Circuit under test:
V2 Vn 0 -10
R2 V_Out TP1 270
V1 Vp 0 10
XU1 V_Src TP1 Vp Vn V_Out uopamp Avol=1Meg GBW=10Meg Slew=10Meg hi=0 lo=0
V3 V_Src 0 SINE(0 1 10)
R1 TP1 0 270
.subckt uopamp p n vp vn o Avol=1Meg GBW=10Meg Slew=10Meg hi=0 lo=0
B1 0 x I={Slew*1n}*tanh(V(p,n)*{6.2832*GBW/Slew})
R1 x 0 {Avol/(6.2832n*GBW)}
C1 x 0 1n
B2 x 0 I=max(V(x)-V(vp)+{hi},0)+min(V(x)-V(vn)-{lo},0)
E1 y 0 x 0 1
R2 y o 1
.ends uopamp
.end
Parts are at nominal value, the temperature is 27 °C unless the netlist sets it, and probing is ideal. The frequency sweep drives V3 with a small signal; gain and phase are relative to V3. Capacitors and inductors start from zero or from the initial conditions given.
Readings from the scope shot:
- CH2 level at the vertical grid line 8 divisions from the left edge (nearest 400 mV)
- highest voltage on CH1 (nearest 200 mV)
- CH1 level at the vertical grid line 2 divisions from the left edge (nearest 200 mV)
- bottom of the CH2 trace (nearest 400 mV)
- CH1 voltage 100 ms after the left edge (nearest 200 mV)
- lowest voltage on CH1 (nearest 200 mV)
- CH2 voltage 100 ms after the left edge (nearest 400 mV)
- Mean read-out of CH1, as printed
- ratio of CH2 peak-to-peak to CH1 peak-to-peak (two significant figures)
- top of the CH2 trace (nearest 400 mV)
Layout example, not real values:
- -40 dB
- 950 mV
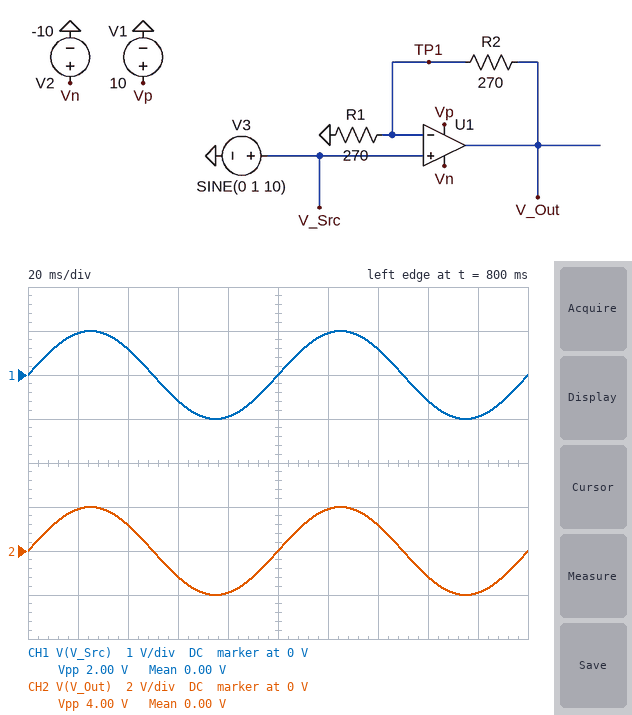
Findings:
- -1.2 V
- 1.0 V
- 600 mV
- -2.0 V
- 0 V
- -1.0 V
- 0 V
- 0.00 V
- 2.0
- 2.0 V
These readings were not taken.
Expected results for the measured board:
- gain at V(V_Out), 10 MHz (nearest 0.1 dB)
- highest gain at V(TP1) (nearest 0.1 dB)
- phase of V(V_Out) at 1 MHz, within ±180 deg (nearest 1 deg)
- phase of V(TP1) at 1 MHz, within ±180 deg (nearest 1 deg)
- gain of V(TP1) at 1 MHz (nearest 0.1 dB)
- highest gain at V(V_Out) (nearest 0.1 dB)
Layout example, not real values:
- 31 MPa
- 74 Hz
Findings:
- -1.0 dB
- 0 dB
- -11 deg
- -11 deg
- -0.2 dB
- 6.0 dB
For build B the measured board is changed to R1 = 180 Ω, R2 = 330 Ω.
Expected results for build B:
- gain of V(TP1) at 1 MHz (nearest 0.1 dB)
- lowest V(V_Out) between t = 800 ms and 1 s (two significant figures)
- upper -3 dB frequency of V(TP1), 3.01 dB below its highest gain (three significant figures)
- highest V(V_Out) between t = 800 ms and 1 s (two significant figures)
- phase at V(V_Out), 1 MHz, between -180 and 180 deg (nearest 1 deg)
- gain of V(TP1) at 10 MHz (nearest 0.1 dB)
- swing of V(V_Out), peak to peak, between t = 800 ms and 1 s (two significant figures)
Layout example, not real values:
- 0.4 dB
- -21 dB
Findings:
- -0.3 dB
- -2.8 V
- 3.52 MHz
- 2.8 V
- -16 deg
- -9.6 dB
- 5.7 V
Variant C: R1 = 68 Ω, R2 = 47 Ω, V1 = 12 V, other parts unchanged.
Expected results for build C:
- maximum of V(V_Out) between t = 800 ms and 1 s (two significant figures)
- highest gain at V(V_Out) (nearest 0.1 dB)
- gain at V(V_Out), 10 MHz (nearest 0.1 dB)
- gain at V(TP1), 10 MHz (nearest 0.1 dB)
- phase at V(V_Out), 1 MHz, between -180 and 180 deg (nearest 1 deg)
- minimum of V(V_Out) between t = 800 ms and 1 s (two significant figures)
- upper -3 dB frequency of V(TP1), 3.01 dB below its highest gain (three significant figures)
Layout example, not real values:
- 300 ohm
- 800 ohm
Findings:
- 1.7 V
- 4.6 dB
- -1.4 dB
- -5.9 dB
- -10 deg
- -1.7 V
- 5.86 MHz
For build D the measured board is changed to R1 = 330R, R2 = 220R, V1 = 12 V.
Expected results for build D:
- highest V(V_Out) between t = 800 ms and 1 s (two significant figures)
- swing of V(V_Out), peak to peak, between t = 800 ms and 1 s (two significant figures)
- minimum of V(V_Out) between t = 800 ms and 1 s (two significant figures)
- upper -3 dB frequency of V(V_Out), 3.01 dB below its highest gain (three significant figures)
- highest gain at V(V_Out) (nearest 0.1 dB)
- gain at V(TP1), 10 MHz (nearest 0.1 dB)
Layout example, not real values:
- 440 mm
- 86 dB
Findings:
- 1.7 V
- 3.3 V
- -1.7 V
- 5.99 MHz
- 4.4 dB
- -5.8 dB
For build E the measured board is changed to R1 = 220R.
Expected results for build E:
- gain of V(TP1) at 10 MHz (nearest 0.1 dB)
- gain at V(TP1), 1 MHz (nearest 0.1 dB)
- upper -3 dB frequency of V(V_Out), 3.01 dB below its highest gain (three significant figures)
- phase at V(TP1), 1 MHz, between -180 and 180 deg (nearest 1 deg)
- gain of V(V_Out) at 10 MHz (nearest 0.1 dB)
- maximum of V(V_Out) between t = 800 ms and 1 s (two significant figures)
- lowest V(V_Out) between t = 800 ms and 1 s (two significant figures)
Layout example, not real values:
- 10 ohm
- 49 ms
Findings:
- -7.8 dB
- -0.2 dB
- 4.48 MHz
- -13 deg
- -0.8 dB
- 2.2 V
- -2.2 V
